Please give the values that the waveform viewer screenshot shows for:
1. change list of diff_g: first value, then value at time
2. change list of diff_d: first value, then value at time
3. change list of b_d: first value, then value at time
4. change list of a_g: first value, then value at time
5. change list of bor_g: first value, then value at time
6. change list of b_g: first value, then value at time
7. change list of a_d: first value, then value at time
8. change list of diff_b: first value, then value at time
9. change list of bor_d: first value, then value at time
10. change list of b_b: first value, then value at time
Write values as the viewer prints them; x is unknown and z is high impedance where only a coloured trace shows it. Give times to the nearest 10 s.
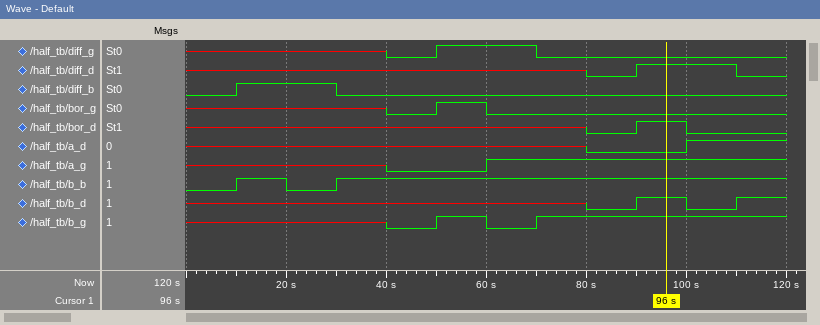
x, 0 at 40 s, 1 at 50 s, 0 at 70 s
x, 0 at 80 s, 1 at 90 s, 0 at 110 s
x, 0 at 80 s, 1 at 90 s, 0 at 100 s, 1 at 110 s
x, 0 at 40 s, 1 at 60 s
x, 0 at 40 s, 1 at 50 s, 0 at 60 s
x, 0 at 40 s, 1 at 50 s, 0 at 60 s, 1 at 70 s
x, 0 at 80 s, 1 at 100 s
0, 1 at 10 s, 0 at 30 s
x, 0 at 80 s, 1 at 90 s, 0 at 100 s
0, 1 at 10 s, 0 at 20 s, 1 at 30 s
